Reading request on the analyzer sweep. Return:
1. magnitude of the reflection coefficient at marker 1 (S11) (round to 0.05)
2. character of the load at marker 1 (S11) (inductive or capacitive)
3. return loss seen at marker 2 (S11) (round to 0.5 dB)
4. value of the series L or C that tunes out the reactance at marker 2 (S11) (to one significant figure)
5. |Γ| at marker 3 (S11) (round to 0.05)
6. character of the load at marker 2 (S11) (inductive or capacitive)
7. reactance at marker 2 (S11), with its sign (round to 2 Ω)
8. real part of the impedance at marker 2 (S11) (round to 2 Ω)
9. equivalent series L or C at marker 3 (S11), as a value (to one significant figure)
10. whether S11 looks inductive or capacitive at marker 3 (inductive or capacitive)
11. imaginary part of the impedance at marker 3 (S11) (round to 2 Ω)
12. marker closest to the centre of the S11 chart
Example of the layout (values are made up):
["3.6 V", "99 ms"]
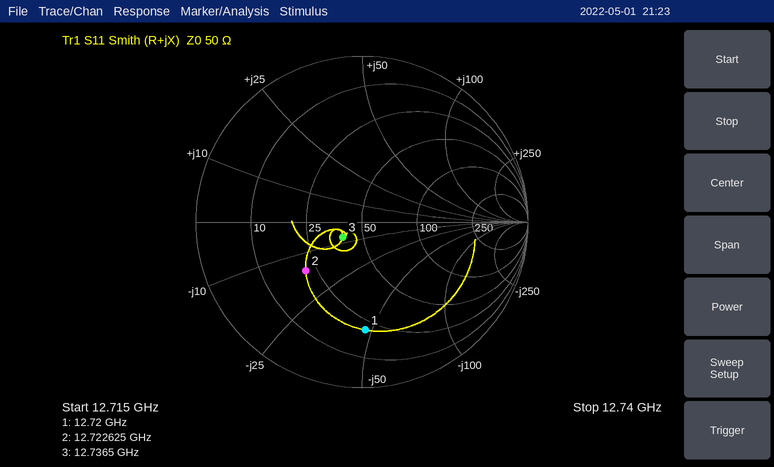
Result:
["0.65", "capacitive", "7.0 dB", "200 pH", "0.15", "capacitive", "-16 Ω", "22 Ω", "2 pF", "capacitive", "-8 Ω", "marker 3"]
